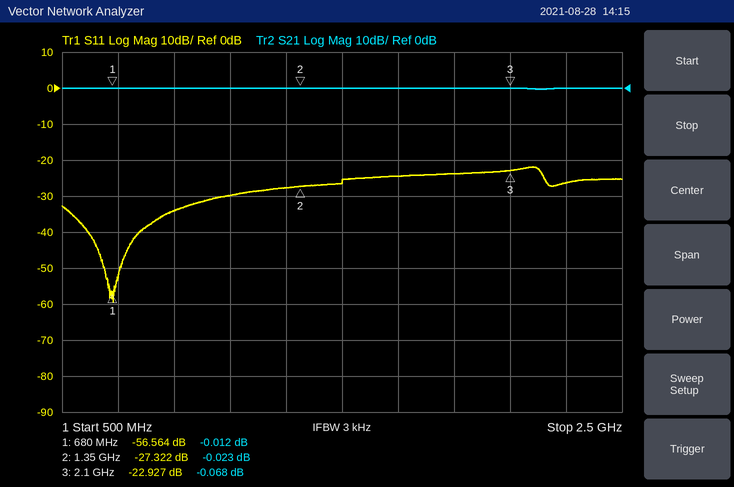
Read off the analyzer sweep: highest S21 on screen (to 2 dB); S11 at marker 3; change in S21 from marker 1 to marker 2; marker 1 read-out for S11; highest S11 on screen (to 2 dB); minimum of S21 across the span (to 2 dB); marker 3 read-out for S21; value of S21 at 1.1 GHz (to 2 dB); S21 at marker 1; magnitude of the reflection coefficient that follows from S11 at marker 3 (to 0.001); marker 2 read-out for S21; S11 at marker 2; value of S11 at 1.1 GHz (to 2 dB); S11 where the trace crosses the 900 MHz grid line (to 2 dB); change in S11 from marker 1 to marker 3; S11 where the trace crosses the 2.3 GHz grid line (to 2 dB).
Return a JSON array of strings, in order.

["0 dB", "-22.927 dB", "-0.011 dB", "-56.564 dB", "-22 dB", "0 dB", "-0.068 dB", "0 dB", "-0.012 dB", "0.071", "-0.023 dB", "-27.322 dB", "-30 dB", "-34 dB", "33.637 dB", "-26 dB"]
